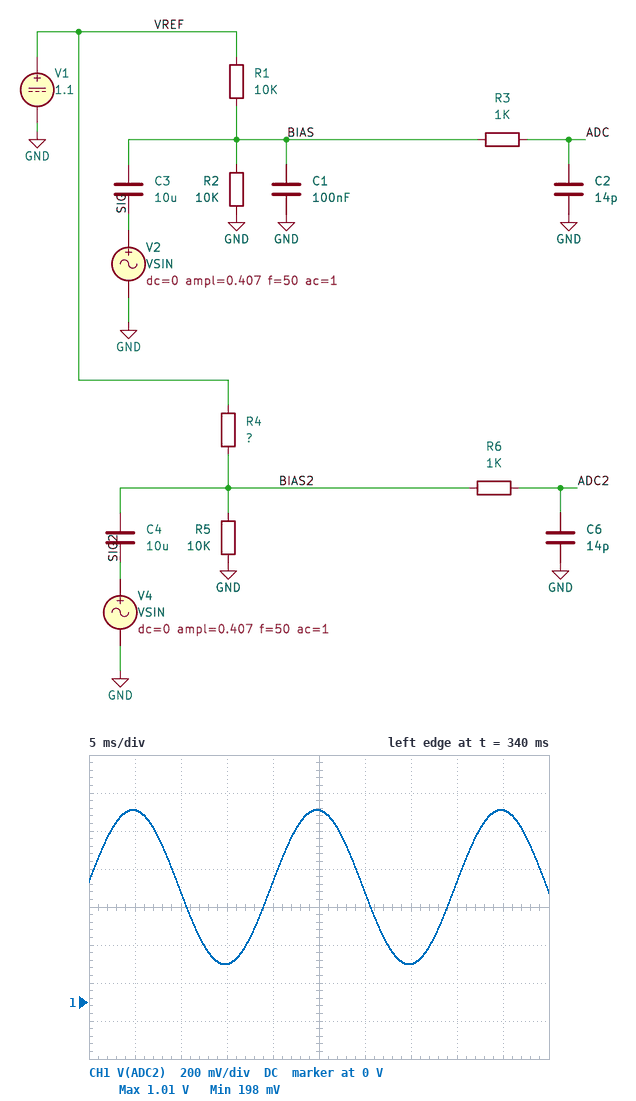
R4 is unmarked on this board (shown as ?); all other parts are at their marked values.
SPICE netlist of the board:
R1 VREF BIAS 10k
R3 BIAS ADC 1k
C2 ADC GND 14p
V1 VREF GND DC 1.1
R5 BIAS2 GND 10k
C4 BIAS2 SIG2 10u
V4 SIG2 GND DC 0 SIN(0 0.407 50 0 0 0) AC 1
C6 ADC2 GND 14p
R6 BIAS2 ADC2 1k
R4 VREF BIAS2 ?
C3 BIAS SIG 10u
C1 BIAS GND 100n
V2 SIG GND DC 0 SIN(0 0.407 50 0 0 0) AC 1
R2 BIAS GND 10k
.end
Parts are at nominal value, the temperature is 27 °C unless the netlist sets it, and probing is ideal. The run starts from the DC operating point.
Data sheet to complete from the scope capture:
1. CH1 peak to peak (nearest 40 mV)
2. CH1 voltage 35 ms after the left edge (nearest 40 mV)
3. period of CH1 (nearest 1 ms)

800 mV
200 mV
20 ms
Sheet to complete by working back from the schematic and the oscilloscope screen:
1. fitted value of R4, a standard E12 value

8.2 kΩ
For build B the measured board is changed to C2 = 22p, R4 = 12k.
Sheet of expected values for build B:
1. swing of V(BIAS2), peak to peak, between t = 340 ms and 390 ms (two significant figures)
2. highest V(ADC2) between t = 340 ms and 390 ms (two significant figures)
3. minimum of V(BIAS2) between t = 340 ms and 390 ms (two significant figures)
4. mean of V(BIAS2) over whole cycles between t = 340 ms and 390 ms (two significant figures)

810 mV
910 mV
94 mV
500 mV
